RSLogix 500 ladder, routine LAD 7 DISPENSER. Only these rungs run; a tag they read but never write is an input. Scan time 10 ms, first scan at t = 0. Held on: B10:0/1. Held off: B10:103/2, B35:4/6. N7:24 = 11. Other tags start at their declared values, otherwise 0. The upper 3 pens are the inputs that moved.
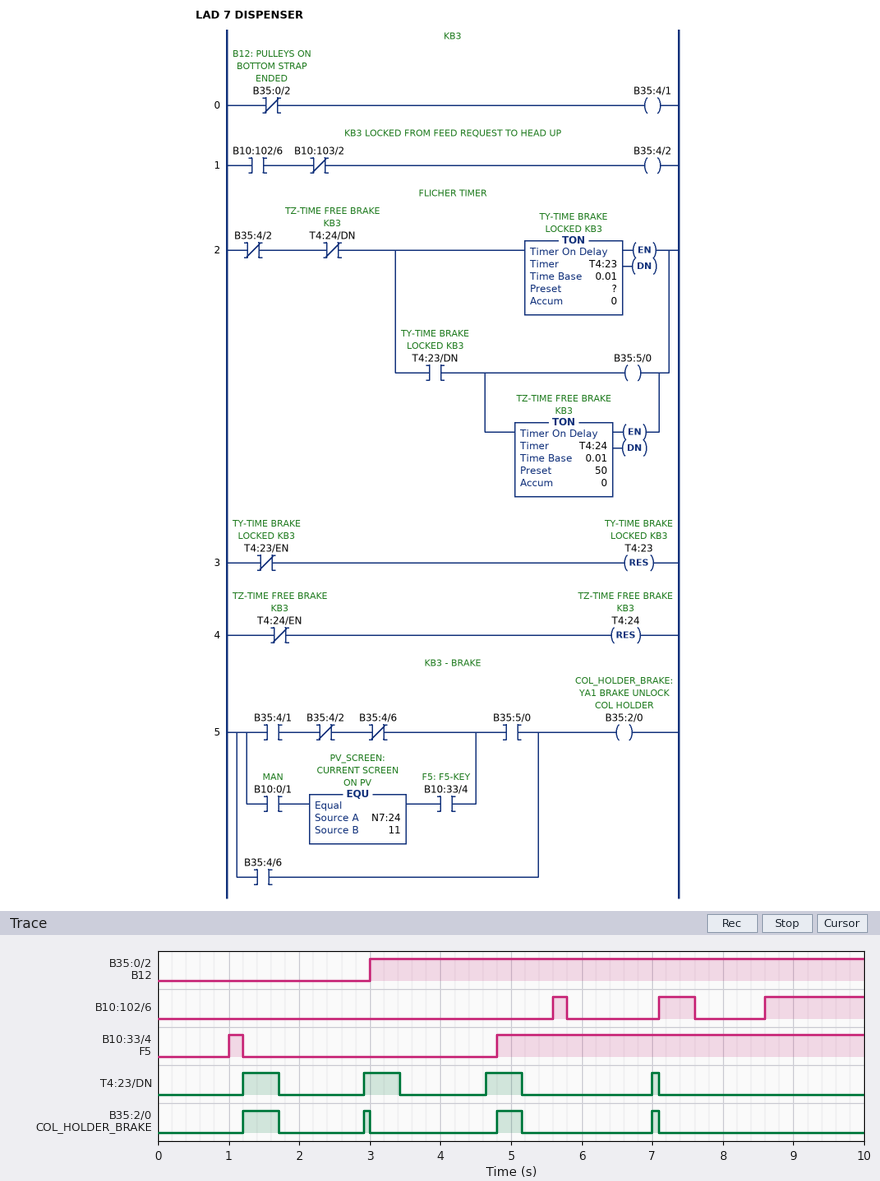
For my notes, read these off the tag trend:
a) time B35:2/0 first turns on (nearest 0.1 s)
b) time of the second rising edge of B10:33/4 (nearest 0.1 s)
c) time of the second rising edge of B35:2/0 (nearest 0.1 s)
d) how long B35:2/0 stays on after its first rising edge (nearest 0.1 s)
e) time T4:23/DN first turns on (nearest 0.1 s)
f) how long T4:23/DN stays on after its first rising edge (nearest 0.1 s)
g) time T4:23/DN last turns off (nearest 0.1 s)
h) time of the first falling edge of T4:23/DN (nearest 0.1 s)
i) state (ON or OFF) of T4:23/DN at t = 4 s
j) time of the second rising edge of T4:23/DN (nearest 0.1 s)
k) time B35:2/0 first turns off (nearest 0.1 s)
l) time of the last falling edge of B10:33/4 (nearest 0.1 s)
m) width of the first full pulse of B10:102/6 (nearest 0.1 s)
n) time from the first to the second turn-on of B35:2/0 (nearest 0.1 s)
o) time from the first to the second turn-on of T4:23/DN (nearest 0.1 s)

1.2 s
4.8 s
2.9 s
0.5 s
1.2 s
0.5 s
7.1 s
1.7 s
OFF
2.9 s
1.7 s
1.2 s
0.2 s
1.7 s
1.7 s
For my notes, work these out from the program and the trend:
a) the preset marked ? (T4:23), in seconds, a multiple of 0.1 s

1.2 s
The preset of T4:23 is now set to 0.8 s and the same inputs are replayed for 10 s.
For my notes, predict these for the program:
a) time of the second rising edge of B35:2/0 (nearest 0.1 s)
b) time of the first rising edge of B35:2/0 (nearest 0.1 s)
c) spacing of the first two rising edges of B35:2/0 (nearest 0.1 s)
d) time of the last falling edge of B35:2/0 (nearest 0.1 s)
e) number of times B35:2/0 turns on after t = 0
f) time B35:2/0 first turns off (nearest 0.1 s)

2.1 s
0.8 s
1.3 s
8.6 s
5
1.3 s
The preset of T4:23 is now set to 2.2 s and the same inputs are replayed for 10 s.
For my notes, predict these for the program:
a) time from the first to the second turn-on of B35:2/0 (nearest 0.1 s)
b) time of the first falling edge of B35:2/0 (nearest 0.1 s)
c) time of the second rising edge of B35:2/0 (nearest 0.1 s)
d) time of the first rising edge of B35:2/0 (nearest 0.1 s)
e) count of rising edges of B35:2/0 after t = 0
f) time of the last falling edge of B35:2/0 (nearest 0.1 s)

2.7 s
2.7 s
4.9 s
2.2 s
2
5.4 s
